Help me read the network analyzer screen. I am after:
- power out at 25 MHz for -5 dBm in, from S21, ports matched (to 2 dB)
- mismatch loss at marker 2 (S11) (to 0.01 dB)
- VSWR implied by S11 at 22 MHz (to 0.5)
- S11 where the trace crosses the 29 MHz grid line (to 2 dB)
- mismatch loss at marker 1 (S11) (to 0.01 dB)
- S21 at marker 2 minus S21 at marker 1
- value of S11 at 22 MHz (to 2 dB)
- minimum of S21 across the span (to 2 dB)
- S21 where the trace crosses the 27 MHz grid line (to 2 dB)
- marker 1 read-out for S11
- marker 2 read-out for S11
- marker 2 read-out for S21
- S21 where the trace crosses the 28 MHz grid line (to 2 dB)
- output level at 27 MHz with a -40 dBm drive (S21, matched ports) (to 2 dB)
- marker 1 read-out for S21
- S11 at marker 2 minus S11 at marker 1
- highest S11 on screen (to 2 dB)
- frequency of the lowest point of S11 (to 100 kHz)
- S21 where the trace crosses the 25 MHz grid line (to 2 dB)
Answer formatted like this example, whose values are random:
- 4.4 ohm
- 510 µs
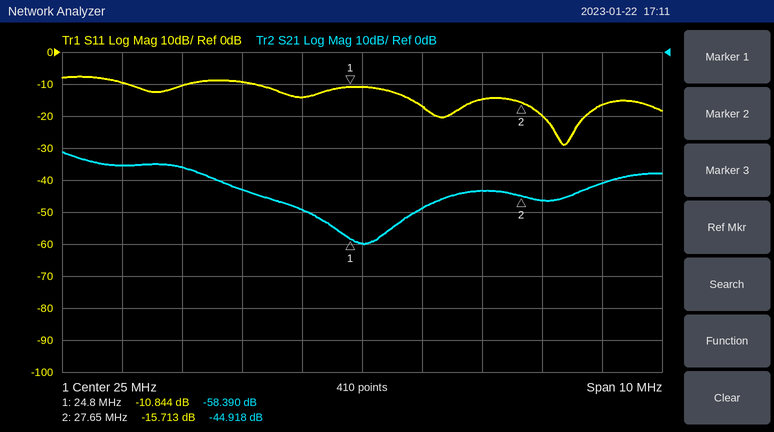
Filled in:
- -64 dBm
- 0.12 dB
- 2.0
- -16 dB
- 0.37 dB
- 13.472 dB
- -10 dB
- -60 dB
- -44 dB
- -10.844 dB
- -15.713 dB
- -44.918 dB
- -46 dB
- -84 dBm
- -58.390 dB
- -4.869 dB
- -8 dB
- 28.4 MHz
- -60 dB
